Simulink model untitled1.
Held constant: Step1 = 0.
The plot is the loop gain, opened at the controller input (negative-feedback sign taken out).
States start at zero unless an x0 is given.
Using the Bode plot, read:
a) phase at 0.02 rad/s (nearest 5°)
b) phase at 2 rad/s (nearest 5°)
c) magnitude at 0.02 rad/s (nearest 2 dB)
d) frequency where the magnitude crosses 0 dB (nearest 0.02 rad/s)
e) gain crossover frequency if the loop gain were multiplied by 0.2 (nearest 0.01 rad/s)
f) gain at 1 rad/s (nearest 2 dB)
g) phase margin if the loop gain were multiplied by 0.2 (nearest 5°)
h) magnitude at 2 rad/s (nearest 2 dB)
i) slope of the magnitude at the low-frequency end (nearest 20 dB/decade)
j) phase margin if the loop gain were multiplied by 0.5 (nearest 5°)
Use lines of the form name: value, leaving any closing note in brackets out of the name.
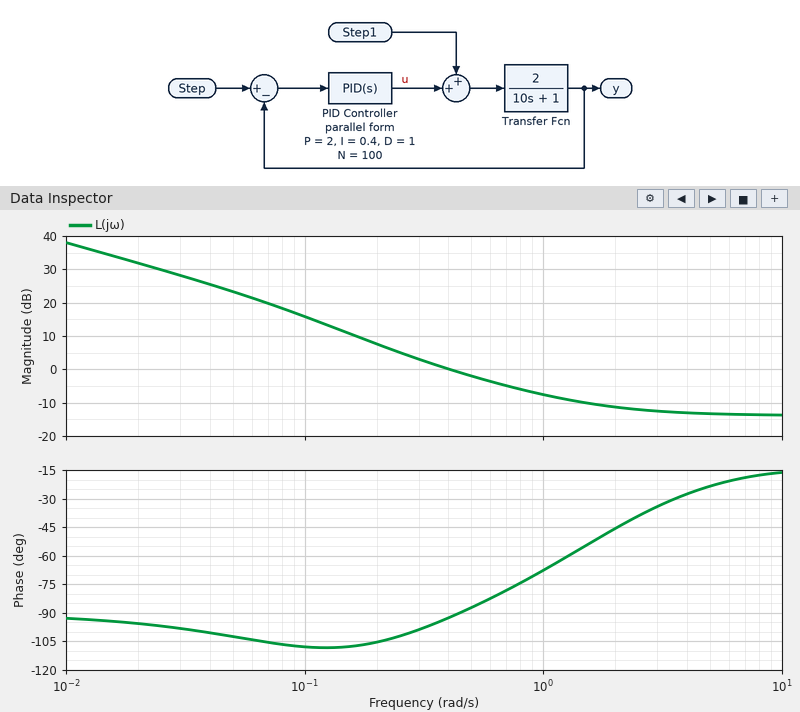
phase at 0.02 rad/s: -95°
phase at 2 rad/s: -45°
magnitude at 0.02 rad/s: 32 dB
frequency where the magnitude crosses 0 dB: 0.40 rad/s
gain crossover frequency if the loop gain were multiplied by 0.2: 0.12 rad/s
gain at 1 rad/s: -8 dB
phase margin if the loop gain were multiplied by 0.2: 70°
magnitude at 2 rad/s: -12 dB
slope of the magnitude at the low-frequency end: -20 dB/decade
phase margin if the loop gain were multiplied by 0.5: 75°
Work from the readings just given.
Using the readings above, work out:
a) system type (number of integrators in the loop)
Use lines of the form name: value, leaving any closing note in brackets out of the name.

system type: 1
